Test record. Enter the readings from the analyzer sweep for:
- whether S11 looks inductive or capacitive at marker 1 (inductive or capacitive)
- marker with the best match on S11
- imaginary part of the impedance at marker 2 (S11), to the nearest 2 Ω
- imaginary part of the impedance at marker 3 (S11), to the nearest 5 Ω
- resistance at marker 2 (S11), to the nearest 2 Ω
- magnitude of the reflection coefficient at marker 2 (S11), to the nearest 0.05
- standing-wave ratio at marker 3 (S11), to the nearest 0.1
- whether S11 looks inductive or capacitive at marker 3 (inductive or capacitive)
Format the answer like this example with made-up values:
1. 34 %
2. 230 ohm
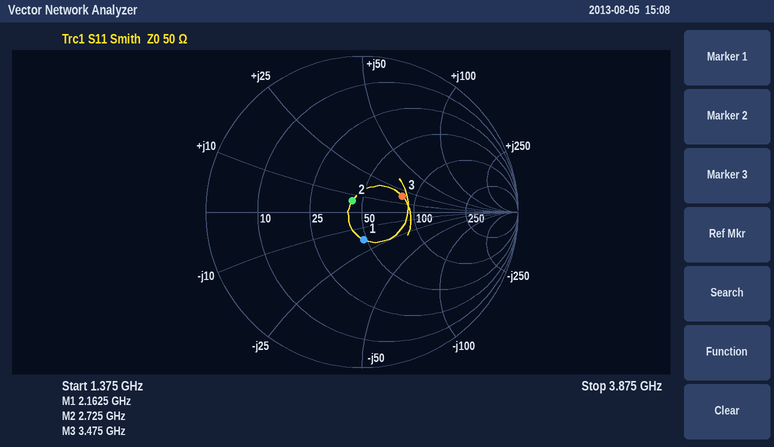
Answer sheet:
1. capacitive
2. marker 2
3. +6 Ω
4. +20 Ω
5. 44 Ω
6. 0.10
7. 1.8
8. inductive
